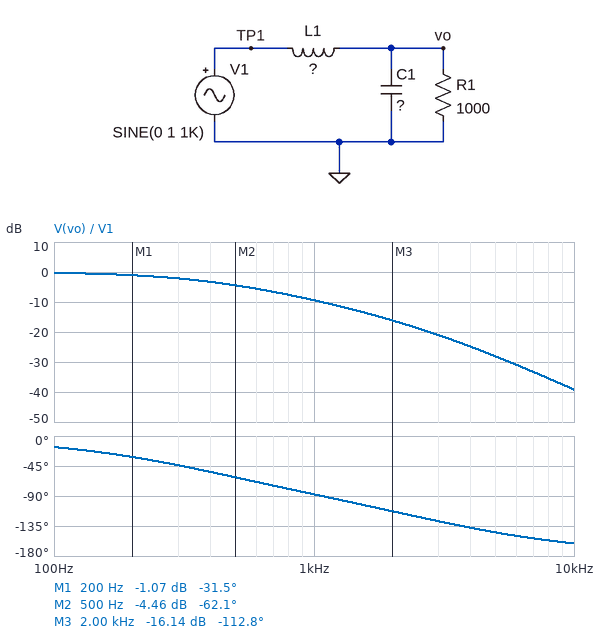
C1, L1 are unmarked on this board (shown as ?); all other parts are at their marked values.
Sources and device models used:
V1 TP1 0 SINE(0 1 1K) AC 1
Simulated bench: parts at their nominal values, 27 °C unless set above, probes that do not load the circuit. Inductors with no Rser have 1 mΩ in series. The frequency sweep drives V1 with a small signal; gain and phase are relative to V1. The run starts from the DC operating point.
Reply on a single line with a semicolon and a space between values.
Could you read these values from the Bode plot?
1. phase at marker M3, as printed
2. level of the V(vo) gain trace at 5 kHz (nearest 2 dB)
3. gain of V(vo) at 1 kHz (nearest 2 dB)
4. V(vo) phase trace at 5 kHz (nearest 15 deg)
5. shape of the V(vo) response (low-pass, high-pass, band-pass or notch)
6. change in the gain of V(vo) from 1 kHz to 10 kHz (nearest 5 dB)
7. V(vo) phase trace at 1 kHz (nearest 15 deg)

-112.8 deg; -28 dB; -10 dB; -150 deg; low-pass; -30 dB; -90 deg
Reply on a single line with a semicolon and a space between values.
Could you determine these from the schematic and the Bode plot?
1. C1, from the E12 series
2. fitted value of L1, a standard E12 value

47 nF; 470 mH
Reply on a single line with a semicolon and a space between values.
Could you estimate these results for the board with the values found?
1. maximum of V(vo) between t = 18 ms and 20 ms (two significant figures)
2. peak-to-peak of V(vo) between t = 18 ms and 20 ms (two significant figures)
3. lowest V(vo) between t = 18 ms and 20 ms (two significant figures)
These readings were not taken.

340 mV; 680 mV; -340 mV
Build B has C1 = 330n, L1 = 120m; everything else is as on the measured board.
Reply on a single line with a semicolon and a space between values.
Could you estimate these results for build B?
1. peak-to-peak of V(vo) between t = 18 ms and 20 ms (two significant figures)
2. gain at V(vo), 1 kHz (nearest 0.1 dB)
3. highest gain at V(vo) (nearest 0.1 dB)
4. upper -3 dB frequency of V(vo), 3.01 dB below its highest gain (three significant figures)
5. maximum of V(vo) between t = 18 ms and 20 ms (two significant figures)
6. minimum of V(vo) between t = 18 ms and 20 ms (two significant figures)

2.1 V; 0.5 dB; 4.8 dB; 944 Hz; 1.1 V; -1.1 V
